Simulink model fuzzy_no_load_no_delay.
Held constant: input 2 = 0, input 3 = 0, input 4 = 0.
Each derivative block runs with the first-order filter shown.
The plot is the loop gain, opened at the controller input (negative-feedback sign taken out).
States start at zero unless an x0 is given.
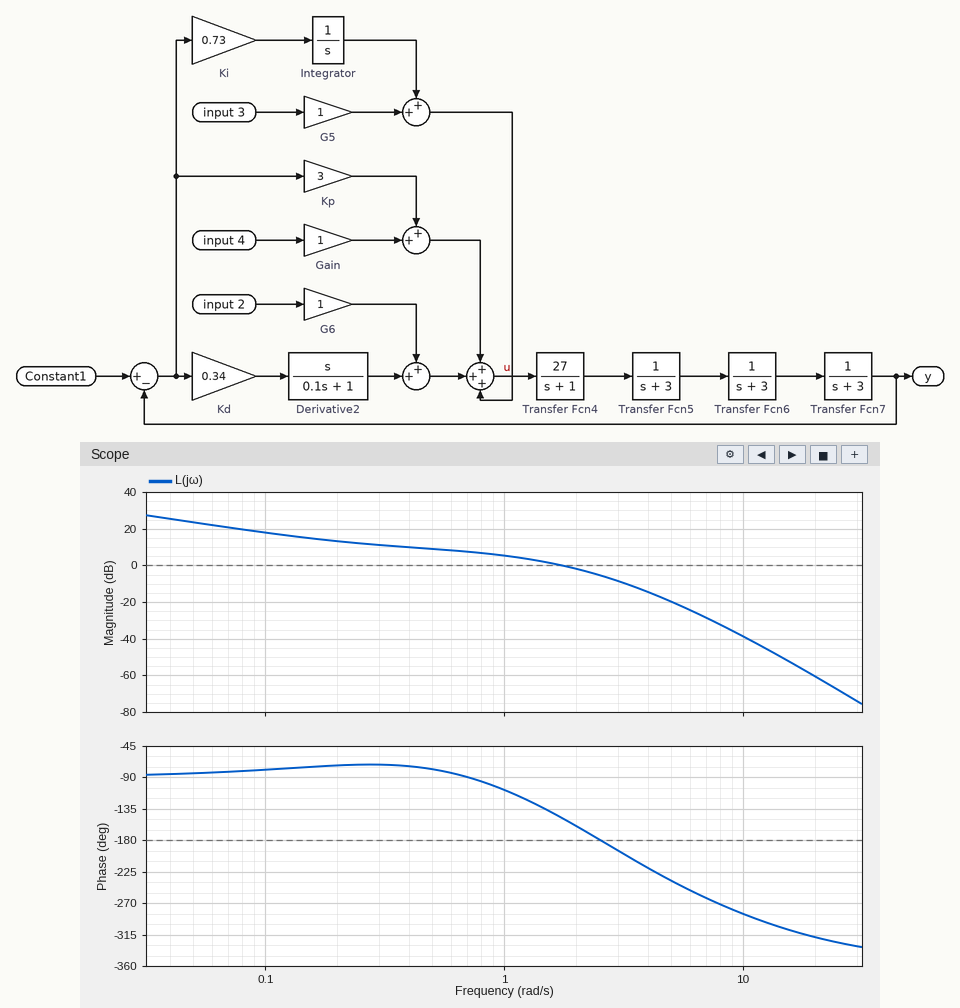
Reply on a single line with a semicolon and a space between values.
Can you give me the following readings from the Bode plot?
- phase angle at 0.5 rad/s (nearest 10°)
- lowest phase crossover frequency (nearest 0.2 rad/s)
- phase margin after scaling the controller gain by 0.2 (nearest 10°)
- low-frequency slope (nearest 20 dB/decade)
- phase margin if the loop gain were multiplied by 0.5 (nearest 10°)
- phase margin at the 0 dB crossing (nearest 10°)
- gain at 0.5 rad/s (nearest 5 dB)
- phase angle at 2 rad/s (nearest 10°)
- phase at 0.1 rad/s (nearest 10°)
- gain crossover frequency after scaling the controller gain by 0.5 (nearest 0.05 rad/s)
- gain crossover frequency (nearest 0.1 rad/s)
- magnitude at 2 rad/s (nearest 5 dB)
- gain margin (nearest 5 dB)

-80°; 2.6 rad/s; 110°; -20 dB/decade; 80°; 30°; 10 dB; -160°; -80°; 0.90 rad/s; 1.7 rad/s; 0 dB; 5 dB
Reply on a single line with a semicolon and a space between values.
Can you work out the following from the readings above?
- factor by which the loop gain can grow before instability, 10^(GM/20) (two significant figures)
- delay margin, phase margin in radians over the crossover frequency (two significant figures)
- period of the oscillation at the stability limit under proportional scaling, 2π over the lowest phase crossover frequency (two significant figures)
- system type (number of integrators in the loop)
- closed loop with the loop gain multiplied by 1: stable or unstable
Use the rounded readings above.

1.8; 0.31 s; 2.4 s; 1; stable
